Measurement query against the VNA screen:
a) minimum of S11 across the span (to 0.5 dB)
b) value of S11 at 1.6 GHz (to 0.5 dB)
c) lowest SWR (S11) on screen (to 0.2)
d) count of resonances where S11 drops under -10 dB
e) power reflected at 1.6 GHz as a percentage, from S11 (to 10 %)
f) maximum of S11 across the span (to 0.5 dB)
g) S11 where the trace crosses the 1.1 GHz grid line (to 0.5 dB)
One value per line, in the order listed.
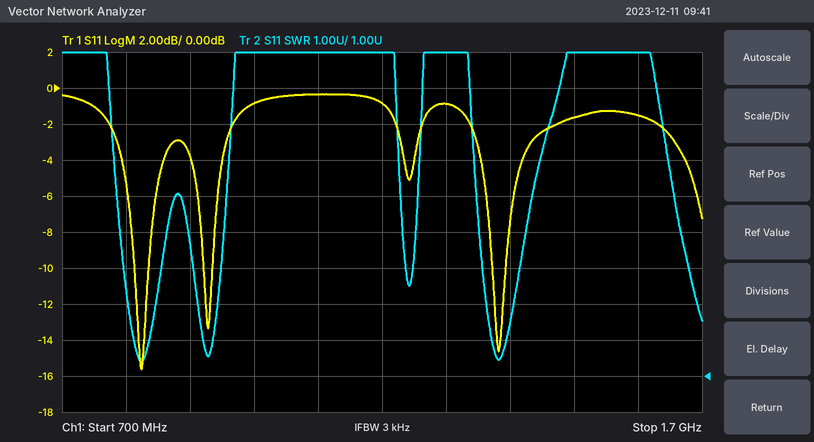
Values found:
-15.5 dB
-1.5 dB
1.4
3
70 %
-0.5 dB
-0.5 dB
